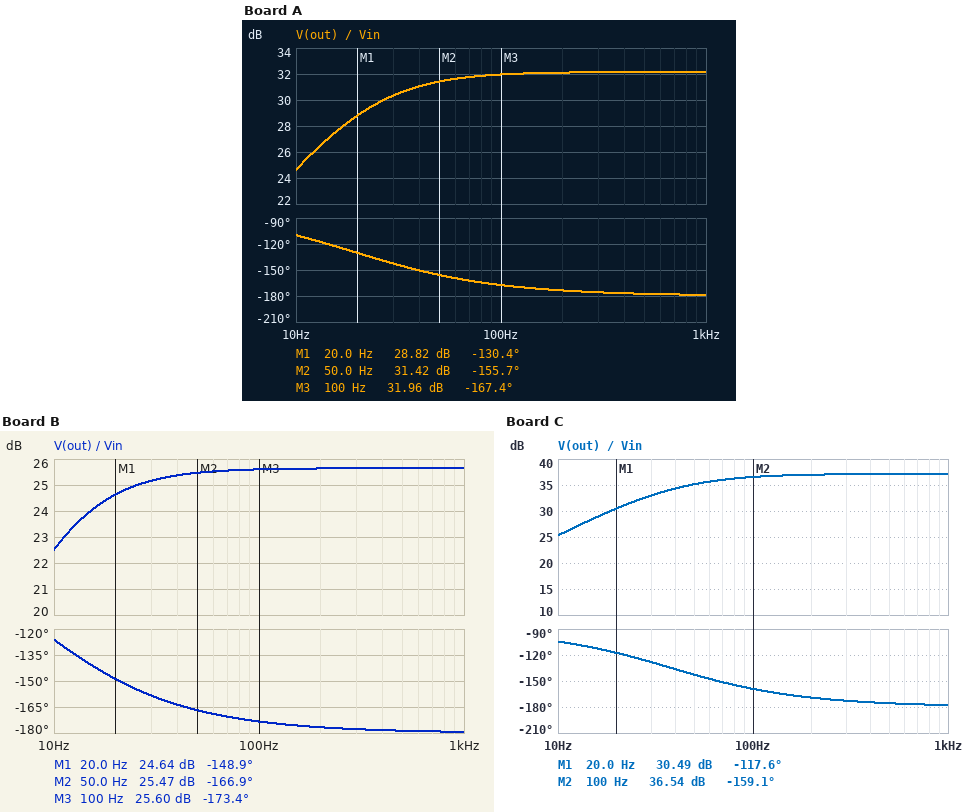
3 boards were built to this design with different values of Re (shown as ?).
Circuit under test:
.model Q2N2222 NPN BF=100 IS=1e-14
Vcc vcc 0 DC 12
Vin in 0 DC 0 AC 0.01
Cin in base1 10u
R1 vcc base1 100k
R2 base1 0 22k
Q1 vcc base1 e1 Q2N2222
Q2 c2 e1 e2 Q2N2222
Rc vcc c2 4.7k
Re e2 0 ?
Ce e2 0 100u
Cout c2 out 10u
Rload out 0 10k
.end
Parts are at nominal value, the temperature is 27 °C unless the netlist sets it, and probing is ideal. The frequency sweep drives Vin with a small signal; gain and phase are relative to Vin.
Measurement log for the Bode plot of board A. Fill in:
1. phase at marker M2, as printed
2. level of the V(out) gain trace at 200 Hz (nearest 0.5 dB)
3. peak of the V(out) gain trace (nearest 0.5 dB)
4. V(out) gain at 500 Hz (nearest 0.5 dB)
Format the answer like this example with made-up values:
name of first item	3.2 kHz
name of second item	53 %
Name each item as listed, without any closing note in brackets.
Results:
phase at marker M2, as printed	-155.7 deg
level of the V(out) gain trace at 200 Hz	32.0 dB
peak of the V(out) gain trace	32.0 dB
V(out) gain at 500 Hz	32.0 dB
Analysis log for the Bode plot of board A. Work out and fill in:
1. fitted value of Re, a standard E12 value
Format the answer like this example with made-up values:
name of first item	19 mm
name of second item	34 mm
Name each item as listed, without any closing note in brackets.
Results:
fitted value of Re, a standard E12 value	1.5 kΩ
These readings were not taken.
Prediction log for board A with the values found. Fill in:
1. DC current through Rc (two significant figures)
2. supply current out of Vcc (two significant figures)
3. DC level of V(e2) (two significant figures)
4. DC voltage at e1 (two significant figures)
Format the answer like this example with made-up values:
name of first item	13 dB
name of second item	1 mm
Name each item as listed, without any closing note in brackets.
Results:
DC current through Rc	660 µA
supply current out of Vcc	760 µA
DC level of V(e2)	990 mV
DC voltage at e1	1.6 V
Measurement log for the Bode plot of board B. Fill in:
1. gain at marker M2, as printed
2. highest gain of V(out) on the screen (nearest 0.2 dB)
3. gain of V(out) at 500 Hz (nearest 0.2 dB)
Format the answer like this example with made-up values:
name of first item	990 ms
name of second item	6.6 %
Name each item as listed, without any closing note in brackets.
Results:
gain at marker M2, as printed	25.47 dB
highest gain of V(out) on the screen	25.6 dB
gain of V(out) at 500 Hz	25.6 dB
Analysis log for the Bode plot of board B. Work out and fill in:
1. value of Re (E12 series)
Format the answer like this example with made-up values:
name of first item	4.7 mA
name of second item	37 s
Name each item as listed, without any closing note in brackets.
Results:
value of Re	3.3 kΩ
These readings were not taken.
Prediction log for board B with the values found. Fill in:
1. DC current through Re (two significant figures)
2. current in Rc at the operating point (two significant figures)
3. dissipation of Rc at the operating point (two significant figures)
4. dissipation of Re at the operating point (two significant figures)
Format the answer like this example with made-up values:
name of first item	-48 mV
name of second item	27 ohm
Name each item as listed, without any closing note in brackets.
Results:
DC current through Re	310 µA
current in Rc at the operating point	310 µA
dissipation of Rc at the operating point	450 µW
dissipation of Re at the operating point	320 µW
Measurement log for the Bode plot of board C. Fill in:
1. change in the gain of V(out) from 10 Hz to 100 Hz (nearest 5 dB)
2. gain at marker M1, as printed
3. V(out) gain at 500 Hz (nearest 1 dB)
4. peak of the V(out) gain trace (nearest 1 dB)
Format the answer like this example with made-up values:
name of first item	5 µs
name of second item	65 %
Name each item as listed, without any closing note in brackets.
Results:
change in the gain of V(out) from 10 Hz to 100 Hz	10 dB
gain at marker M1, as printed	30.49 dB
V(out) gain at 500 Hz	37 dB
peak of the V(out) gain trace	37 dB
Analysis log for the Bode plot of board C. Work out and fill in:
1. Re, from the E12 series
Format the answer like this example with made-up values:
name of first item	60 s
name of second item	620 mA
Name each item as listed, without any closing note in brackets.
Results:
Re, from the E12 series	820 Ω
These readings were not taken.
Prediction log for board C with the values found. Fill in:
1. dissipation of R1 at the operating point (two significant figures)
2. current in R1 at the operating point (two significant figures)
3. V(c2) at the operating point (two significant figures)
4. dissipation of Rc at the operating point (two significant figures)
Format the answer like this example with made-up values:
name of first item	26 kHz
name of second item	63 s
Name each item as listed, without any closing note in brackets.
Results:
dissipation of R1 at the operating point	970 µW
current in R1 at the operating point	98 µA
V(c2) at the operating point	6.5 V
dissipation of Rc at the operating point	6.4 mW
